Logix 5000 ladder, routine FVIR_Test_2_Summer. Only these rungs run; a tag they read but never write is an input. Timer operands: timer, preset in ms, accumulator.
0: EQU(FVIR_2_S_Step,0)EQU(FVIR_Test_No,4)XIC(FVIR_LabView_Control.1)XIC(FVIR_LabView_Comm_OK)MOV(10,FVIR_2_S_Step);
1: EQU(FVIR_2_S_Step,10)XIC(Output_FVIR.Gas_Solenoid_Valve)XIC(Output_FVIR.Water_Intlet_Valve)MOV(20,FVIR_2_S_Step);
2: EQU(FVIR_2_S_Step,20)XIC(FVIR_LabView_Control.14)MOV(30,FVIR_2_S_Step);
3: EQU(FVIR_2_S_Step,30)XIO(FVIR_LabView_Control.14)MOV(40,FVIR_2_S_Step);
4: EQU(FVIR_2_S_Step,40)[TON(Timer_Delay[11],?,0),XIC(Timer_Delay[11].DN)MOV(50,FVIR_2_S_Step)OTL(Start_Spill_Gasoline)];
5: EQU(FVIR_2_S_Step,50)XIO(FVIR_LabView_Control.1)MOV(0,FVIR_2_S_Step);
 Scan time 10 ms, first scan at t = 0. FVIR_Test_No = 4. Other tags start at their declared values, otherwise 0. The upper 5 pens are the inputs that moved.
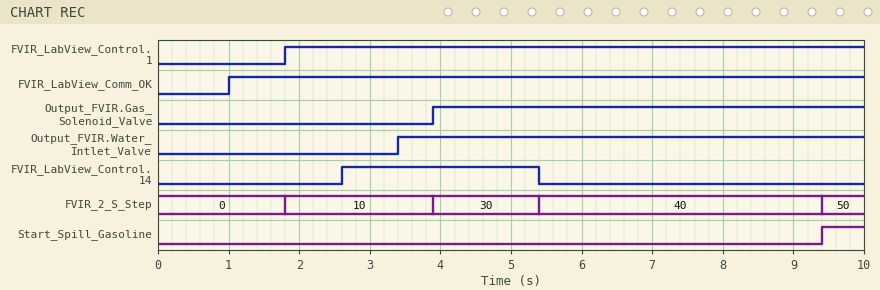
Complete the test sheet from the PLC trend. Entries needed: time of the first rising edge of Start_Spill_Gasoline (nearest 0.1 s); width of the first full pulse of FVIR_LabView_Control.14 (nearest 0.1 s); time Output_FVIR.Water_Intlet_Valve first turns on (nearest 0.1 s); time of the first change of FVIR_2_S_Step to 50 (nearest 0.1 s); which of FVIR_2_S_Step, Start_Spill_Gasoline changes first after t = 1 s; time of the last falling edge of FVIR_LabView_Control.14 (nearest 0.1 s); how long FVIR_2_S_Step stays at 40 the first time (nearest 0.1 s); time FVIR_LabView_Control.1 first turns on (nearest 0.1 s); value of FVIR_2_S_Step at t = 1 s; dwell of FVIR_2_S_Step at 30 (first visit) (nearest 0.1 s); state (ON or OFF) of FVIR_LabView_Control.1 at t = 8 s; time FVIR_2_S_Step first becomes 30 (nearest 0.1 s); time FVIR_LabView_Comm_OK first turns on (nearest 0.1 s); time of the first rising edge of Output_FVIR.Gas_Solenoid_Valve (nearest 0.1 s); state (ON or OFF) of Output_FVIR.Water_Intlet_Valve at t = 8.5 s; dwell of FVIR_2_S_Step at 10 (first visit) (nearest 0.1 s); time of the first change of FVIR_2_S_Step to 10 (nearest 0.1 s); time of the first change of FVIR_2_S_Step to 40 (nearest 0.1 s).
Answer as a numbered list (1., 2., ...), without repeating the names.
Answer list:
1. 9.4 s
2. 2.8 s
3. 3.4 s
4. 9.4 s
5. FVIR_2_S_Step
6. 5.4 s
7. 4.0 s
8. 1.8 s
9. 0
10. 1.5 s
11. ON
12. 3.9 s
13. 1.0 s
14. 3.9 s
15. ON
16. 2.1 s
17. 1.8 s
18. 5.4 s
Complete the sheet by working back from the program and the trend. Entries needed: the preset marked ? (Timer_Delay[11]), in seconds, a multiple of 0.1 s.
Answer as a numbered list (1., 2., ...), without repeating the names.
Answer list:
1. 4.0 s
